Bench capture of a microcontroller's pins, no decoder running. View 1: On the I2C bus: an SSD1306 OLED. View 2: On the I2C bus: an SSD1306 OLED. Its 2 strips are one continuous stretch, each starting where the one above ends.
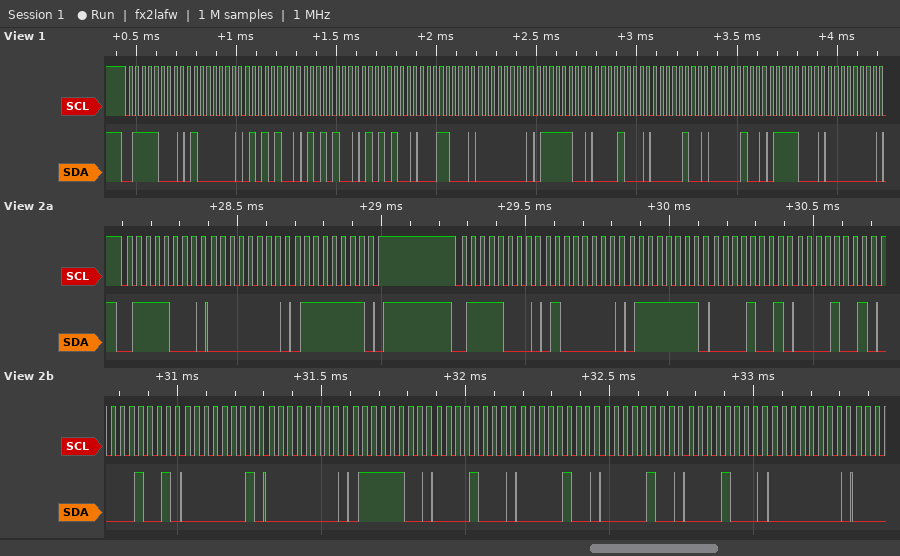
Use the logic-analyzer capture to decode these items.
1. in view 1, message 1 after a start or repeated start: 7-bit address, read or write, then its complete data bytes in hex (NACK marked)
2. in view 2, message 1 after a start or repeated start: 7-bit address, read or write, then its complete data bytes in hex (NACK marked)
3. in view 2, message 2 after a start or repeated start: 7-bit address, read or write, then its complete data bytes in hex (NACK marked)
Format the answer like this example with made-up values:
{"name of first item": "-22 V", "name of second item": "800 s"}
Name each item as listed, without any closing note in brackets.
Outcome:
{"in view 1, message 1 after a start or repeated start: 7-bit address, read or write, then its complete data bytes in hex": "0x3C write: 40 54 54 54 18 00 7C 08 04 04 78 00", "in view 2, message 1 after a start or repeated start: 7-bit address, read or write, then its complete data bytes in hex": "0x3C write: 00 7F", "in view 2, message 2 after a start or repeated start: 7-bit address, read or write, then its complete data bytes in hex": "0x3C write: 40 7F 09 09 09 01 00 7C 08 04 04 08 00"}
